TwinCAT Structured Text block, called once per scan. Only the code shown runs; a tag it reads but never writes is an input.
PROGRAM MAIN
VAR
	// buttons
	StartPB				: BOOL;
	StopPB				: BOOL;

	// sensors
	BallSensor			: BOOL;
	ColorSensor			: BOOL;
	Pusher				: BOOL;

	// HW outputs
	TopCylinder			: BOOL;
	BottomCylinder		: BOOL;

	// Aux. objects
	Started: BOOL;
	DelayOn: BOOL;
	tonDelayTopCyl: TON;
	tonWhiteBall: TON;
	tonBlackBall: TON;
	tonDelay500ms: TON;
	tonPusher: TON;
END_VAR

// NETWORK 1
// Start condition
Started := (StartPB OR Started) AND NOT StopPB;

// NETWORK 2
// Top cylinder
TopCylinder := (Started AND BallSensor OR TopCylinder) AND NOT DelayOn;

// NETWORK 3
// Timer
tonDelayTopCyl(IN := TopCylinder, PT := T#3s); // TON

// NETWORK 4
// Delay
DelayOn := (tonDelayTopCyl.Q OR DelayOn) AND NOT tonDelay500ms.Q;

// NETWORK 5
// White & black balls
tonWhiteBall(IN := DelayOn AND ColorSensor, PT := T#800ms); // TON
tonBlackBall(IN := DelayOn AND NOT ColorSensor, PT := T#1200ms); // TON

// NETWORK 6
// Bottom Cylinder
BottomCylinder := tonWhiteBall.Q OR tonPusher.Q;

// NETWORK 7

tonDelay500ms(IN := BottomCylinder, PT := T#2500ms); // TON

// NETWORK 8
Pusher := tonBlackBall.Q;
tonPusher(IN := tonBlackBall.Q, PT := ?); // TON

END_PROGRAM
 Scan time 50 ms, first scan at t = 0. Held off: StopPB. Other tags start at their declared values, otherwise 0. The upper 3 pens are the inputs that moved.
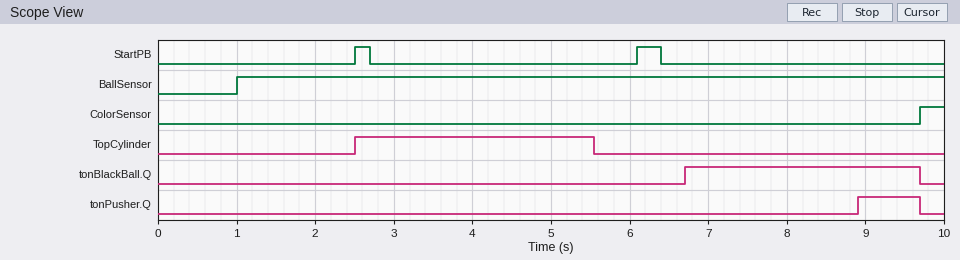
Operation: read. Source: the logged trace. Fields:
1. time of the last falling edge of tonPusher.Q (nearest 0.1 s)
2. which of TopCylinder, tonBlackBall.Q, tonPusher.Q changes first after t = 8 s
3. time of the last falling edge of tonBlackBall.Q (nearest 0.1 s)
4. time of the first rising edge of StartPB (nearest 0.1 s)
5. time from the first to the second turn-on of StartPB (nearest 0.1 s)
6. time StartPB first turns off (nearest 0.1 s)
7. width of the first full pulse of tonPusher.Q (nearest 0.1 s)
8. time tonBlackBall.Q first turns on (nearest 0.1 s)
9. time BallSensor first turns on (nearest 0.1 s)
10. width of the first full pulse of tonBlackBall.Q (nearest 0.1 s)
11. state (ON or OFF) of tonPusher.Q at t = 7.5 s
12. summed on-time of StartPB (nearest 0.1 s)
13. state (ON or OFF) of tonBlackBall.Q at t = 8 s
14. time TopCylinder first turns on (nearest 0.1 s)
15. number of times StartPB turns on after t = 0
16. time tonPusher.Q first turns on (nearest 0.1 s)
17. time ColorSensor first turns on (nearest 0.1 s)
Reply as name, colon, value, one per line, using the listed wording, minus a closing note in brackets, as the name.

time of the last falling edge of tonPusher.Q: 9.7 s
which of TopCylinder, tonBlackBall.Q, tonPusher.Q changes first after t = 8 s: tonPusher.Q
time of the last falling edge of tonBlackBall.Q: 9.7 s
time of the first rising edge of StartPB: 2.5 s
time from the first to the second turn-on of StartPB: 3.6 s
time StartPB first turns off: 2.7 s
width of the first full pulse of tonPusher.Q: 0.8 s
time tonBlackBall.Q first turns on: 6.7 s
time BallSensor first turns on: 1.0 s
width of the first full pulse of tonBlackBall.Q: 3.0 s
state (ON or OFF) of tonPusher.Q at t = 7.5 s: OFF
summed on-time of StartPB: 0.5 s
state (ON or OFF) of tonBlackBall.Q at t = 8 s: ON
time TopCylinder first turns on: 2.5 s
number of times StartPB turns on after t = 0: 2
time tonPusher.Q first turns on: 8.9 s
time ColorSensor first turns on: 9.7 s
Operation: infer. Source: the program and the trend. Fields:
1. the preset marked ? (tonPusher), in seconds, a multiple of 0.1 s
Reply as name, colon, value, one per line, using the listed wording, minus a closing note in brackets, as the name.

the preset marked ? (tonPusher), in seconds, a multiple of 0.1 s: 2.2 s
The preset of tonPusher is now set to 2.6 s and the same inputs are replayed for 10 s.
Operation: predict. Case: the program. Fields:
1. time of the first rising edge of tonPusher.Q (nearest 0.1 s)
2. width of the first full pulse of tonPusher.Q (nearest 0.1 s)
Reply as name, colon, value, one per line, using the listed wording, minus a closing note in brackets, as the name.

time of the first rising edge of tonPusher.Q: 9.3 s
width of the first full pulse of tonPusher.Q: 0.4 s
